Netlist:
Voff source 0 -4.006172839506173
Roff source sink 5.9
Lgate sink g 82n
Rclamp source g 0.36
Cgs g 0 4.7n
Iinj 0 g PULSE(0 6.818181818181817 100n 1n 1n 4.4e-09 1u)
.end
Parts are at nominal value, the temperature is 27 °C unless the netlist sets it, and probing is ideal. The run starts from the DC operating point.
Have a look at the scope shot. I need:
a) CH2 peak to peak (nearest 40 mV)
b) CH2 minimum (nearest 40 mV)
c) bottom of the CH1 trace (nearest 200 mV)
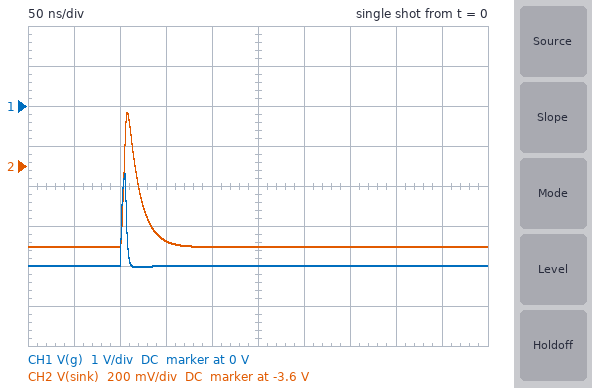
680 mV
-4.00 V
-4.0 V
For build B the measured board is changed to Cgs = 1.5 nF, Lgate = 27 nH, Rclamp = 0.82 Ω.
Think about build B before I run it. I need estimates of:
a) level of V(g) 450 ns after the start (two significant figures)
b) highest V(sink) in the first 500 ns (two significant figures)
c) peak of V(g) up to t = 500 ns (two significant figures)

-4.0 V
-780 mV
1.2 V
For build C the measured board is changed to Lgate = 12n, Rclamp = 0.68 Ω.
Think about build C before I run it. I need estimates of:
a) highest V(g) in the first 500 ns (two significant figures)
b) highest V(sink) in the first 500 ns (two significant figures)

-490 mV
-1.1 V
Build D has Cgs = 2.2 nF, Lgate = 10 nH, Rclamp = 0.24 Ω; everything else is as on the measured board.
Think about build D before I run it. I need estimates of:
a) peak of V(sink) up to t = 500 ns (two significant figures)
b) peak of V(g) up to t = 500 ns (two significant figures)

-2.5 V
-2.4 V
